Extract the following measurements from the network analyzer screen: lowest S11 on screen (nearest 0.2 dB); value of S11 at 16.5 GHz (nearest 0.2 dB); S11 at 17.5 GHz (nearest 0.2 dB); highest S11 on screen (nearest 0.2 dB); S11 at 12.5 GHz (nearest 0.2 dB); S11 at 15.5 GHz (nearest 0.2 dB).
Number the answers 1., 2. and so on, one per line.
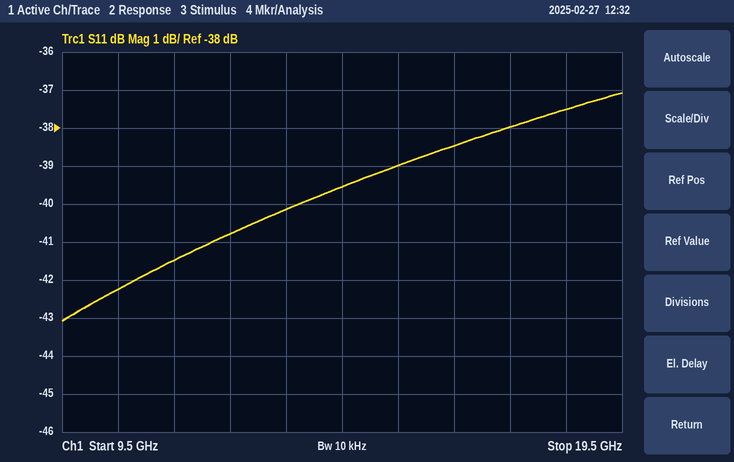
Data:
1. -43.0 dB
2. -38.4 dB
3. -38.0 dB
4. -37.0 dB
5. -40.8 dB
6. -39.0 dB
